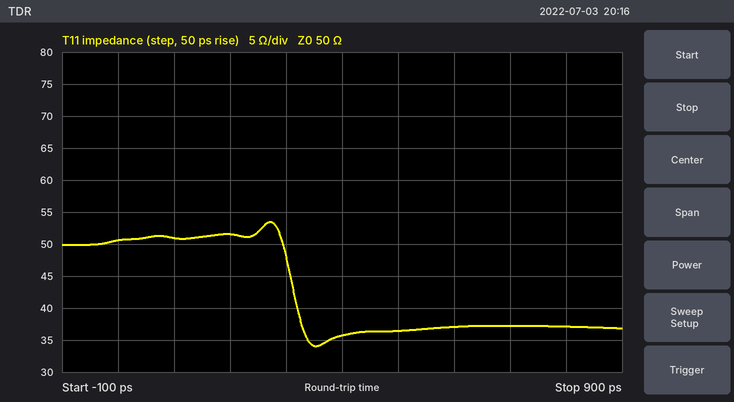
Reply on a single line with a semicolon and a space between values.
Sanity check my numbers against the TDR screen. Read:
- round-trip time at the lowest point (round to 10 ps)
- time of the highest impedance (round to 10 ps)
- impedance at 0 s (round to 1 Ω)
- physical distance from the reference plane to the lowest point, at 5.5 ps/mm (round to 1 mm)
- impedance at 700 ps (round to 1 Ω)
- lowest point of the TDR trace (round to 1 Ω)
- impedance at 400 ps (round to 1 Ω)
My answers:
350 ps; 270 ps; 51 Ω; 32 mm; 37 Ω; 34 Ω; 36 Ω
